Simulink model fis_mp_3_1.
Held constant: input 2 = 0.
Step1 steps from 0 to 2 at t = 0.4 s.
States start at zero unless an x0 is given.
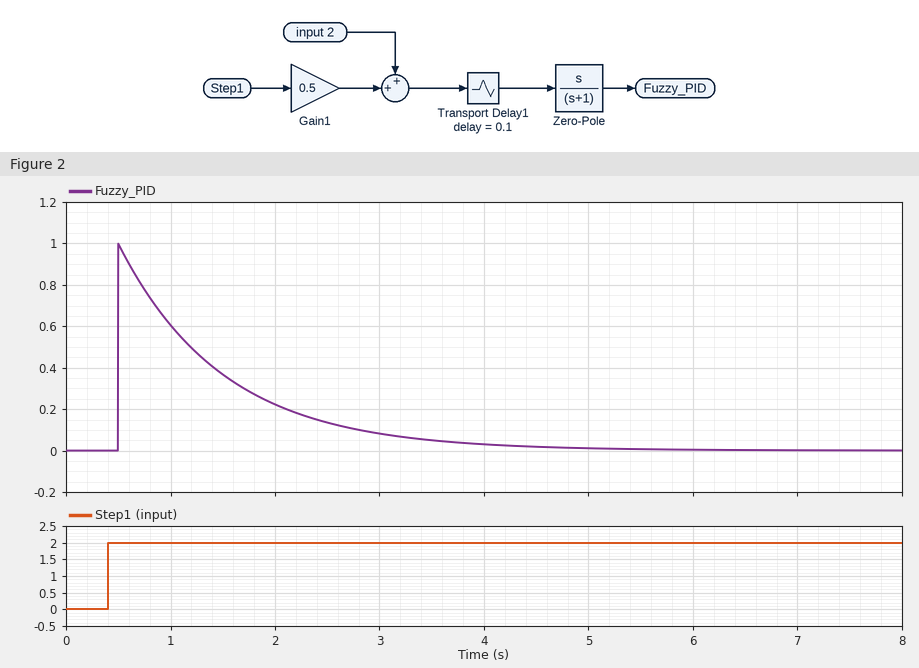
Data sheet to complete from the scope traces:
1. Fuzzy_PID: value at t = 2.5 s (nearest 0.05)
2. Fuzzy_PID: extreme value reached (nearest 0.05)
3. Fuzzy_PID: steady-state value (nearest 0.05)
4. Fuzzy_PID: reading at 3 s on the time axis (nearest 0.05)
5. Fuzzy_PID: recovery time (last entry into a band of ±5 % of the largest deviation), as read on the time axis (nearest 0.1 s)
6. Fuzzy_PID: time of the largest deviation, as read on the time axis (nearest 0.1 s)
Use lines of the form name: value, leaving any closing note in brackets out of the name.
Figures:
Fuzzy_PID: value at t = 2.5 s: 0.15
Fuzzy_PID: extreme value reached: 1.00
Fuzzy_PID: steady-state value: 0.00
Fuzzy_PID: reading at 3 s on the time axis: 0.10
Fuzzy_PID: recovery time (last entry into a band of ±5 % of the largest deviation), as read on the time axis: 3.5 s
Fuzzy_PID: time of the largest deviation, as read on the time axis: 0.5 s
